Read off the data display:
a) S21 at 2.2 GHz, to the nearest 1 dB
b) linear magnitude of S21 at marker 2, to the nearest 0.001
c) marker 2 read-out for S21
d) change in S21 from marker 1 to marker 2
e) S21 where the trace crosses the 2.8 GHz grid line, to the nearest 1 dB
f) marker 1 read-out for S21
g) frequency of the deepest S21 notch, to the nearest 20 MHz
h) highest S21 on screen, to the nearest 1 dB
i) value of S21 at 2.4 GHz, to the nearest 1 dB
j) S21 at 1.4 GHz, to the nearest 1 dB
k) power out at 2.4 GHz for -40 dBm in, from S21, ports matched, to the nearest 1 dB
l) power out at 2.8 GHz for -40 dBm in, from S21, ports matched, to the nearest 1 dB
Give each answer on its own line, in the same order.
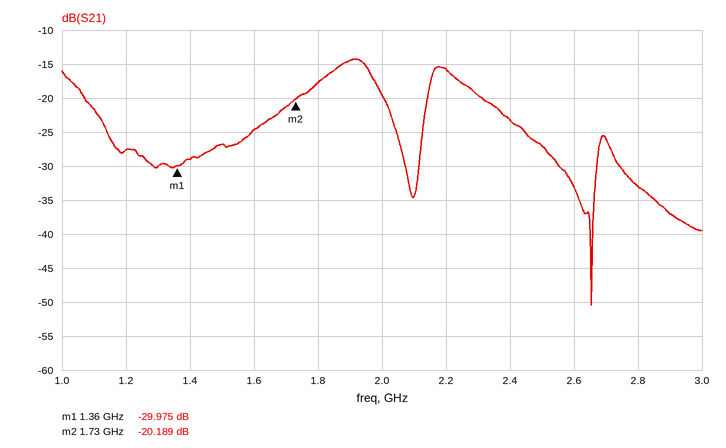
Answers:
-16 dB
0.098
-20.189 dB
9.786 dB
-33 dB
-29.975 dB
2.66 GHz
-14 dB
-23 dB
-29 dB
-63 dBm
-73 dBm
